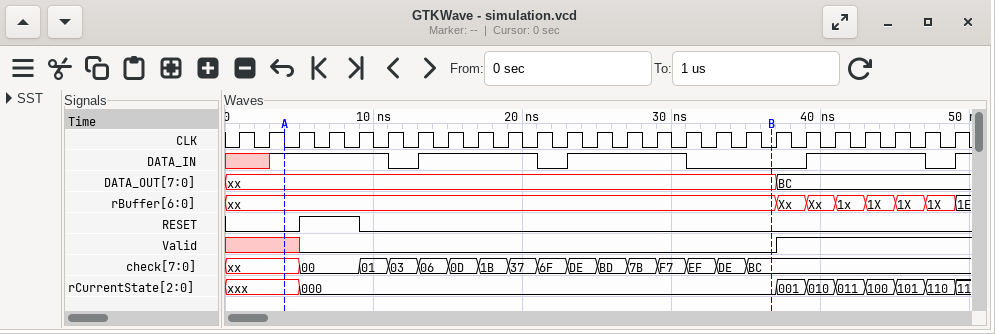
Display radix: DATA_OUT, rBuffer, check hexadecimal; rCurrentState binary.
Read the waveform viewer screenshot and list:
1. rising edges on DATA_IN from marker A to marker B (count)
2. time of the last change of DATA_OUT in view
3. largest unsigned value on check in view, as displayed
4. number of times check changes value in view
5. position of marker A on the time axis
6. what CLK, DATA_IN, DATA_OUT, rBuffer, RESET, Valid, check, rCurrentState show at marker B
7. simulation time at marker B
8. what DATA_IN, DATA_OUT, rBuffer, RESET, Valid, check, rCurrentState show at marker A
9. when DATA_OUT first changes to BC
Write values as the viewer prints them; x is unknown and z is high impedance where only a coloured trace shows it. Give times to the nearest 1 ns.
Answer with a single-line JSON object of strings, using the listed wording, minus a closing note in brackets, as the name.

{"rising edges on DATA_IN from marker A to marker B": "2", "time of the last change of DATA_OUT in view": "37 ns", "largest unsigned value on check in view, as displayed": "F7", "number of times check changes value in view": "15", "position of marker A on the time axis": "4 ns", "what CLK, DATA_IN, DATA_OUT, rBuffer, RESET, Valid, check, rCurrentState show at marker B": "CLK=0, DATA_IN=0, DATA_OUT=xx, rBuffer=xx, RESET=0, Valid=0, check=BC, rCurrentState=000", "simulation time at marker B": "37 ns", "what DATA_IN, DATA_OUT, rBuffer, RESET, Valid, check, rCurrentState show at marker A": "DATA_IN=1, DATA_OUT=xx, rBuffer=xx, RESET=0, Valid=x, check=xx, rCurrentState=xxx", "when DATA_OUT first changes to BC": "37 ns"}
